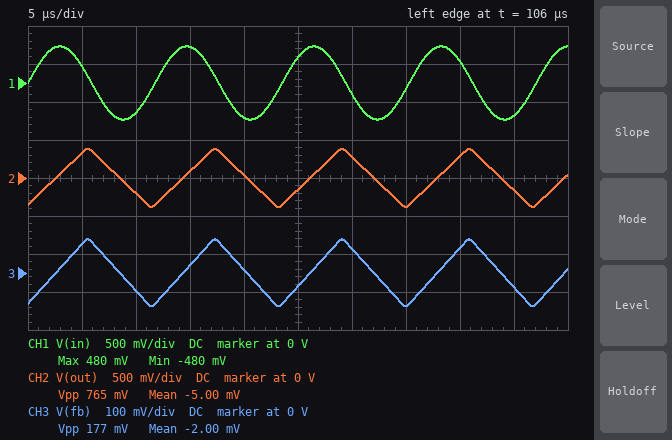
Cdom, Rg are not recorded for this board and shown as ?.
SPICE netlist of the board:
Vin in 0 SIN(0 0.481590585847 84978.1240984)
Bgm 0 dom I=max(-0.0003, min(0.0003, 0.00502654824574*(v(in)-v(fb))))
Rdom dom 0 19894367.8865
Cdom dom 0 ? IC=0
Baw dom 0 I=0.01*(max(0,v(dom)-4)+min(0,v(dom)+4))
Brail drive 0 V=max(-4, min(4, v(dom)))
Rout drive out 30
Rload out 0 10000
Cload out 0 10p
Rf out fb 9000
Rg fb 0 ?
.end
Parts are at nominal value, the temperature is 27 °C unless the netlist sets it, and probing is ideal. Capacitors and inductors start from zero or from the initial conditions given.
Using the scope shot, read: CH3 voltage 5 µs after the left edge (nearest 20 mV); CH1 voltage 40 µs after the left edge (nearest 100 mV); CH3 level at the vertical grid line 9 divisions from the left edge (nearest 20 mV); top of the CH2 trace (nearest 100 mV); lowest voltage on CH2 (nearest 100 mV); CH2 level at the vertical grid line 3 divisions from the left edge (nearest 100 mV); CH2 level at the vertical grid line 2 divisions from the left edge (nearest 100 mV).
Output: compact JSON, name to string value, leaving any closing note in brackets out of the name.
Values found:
{"CH3 voltage 5 µs after the left edge": "80 mV", "CH1 voltage 40 µs after the left edge": "300 mV", "CH3 level at the vertical grid line 9 divisions from the left edge": "-40 mV", "top of the CH2 trace": "400 mV", "lowest voltage on CH2": "-400 mV", "CH2 level at the vertical grid line 3 divisions from the left edge": "100 mV", "CH2 level at the vertical grid line 2 divisions from the left edge": "-200 mV"}
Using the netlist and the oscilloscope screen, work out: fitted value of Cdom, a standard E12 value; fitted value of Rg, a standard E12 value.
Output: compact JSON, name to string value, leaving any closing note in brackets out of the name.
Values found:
{"fitted value of Cdom, a standard E12 value": "2.2 nF", "fitted value of Rg, a standard E12 value": "2.7 kΩ"}
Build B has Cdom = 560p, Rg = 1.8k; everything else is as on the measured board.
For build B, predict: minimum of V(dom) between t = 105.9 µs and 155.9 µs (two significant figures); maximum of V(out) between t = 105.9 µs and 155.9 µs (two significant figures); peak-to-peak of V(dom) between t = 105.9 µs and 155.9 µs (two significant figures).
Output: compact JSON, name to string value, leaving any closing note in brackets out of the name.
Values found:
{"minimum of V(dom) between t = 105.9 µs and 155.9 µs": "-1.5 V", "maximum of V(out) between t = 105.9 µs and 155.9 µs": "1.5 V", "peak-to-peak of V(dom) between t = 105.9 µs and 155.9 µs": "3.0 V"}
